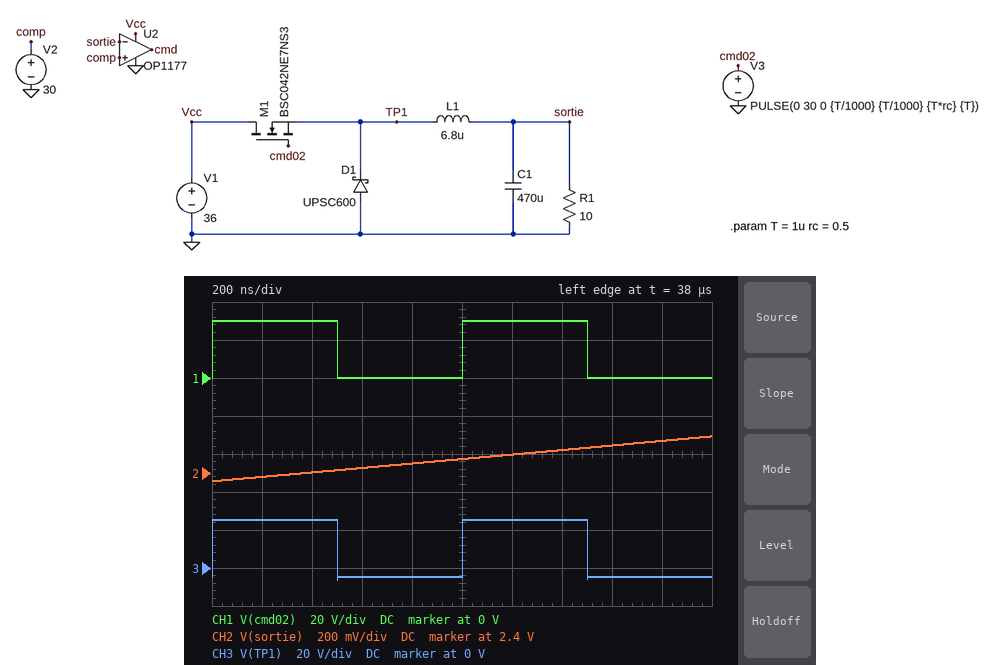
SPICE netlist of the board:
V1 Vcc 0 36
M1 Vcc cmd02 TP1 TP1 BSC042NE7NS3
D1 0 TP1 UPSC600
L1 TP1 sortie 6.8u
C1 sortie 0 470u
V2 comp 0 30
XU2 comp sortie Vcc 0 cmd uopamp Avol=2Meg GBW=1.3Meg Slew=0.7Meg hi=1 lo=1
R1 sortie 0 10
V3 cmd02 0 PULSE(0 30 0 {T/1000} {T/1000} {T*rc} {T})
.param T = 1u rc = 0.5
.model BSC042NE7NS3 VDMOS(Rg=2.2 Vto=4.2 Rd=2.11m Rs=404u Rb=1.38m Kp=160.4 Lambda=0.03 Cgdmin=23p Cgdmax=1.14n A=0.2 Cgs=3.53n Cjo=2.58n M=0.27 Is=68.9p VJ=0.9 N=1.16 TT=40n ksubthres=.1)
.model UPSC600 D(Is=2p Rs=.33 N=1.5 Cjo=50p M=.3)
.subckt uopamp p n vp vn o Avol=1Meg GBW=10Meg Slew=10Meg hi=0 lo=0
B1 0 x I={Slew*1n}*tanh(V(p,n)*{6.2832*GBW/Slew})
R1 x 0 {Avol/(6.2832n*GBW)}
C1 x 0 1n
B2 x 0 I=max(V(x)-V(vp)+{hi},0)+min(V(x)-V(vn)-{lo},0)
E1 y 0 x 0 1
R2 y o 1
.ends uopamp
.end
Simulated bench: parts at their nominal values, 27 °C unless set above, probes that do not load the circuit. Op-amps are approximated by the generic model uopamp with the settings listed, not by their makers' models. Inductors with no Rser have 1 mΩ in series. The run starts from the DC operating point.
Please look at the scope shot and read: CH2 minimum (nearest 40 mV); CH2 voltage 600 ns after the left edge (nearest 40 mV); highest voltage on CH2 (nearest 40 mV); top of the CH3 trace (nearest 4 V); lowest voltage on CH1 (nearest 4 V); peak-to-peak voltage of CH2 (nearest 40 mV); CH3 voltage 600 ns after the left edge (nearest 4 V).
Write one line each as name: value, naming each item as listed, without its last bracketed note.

CH2 minimum: 2.36 V
CH2 voltage 600 ns after the left edge: 2.44 V
highest voltage on CH2: 2.60 V
top of the CH3 trace: 24 V
lowest voltage on CH1: 0 V
peak-to-peak voltage of CH2: 240 mV
CH3 voltage 600 ns after the left edge: -4 V
